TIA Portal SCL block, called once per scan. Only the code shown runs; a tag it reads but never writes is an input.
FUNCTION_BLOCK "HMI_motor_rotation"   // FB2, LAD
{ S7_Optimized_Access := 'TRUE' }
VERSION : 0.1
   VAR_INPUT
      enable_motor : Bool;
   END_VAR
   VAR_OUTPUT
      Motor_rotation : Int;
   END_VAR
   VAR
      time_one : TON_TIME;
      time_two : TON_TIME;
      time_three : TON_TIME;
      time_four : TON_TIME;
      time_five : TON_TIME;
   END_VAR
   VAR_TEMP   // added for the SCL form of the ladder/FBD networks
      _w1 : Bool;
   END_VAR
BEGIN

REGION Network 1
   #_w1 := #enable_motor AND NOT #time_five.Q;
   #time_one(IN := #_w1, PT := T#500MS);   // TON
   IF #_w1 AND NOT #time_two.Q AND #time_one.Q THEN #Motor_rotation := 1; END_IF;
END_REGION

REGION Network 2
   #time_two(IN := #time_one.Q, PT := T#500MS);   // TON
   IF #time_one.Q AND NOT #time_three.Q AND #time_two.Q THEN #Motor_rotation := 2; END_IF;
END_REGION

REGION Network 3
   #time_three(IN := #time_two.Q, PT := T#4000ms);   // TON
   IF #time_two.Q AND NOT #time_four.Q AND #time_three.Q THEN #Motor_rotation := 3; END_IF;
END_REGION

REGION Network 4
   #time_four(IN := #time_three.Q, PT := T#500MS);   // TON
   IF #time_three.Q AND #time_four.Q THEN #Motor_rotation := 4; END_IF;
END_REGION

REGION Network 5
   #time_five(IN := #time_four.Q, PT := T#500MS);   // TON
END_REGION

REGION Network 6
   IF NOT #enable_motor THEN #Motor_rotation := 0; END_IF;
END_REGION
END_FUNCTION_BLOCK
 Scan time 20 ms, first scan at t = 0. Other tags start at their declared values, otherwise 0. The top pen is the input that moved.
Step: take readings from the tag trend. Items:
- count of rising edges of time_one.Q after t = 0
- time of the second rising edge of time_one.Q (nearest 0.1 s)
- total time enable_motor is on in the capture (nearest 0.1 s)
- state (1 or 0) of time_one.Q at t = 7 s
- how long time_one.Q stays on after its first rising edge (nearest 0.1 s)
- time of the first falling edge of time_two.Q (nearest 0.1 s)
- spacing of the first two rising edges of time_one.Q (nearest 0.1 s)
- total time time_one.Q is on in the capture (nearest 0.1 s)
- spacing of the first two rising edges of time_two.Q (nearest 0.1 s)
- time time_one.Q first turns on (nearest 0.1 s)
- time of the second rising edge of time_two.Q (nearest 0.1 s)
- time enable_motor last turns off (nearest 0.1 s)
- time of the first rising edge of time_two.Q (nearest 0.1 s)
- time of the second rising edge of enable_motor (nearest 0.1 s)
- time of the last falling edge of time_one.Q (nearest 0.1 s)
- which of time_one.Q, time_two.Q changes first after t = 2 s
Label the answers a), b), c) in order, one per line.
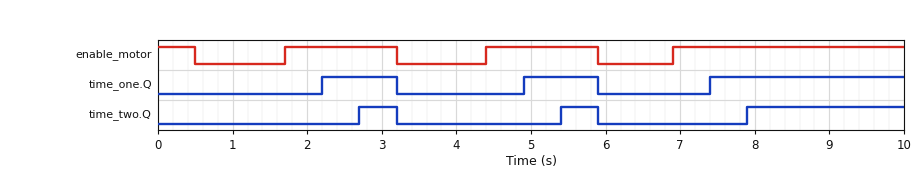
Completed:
a) 3
b) 4.9 s
c) 6.6 s
d) 0
e) 1.0 s
f) 3.2 s
g) 2.7 s
h) 4.6 s
i) 2.7 s
j) 2.2 s
k) 5.4 s
l) 5.9 s
m) 2.7 s
n) 4.4 s
o) 5.9 s
p) time_one.Q
